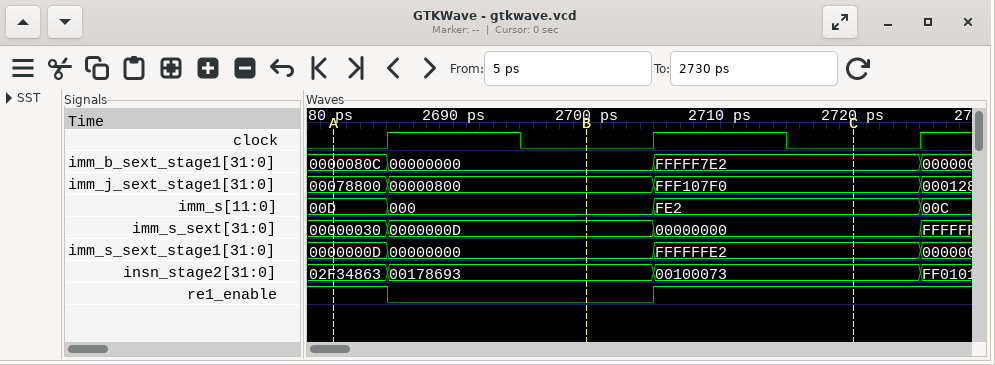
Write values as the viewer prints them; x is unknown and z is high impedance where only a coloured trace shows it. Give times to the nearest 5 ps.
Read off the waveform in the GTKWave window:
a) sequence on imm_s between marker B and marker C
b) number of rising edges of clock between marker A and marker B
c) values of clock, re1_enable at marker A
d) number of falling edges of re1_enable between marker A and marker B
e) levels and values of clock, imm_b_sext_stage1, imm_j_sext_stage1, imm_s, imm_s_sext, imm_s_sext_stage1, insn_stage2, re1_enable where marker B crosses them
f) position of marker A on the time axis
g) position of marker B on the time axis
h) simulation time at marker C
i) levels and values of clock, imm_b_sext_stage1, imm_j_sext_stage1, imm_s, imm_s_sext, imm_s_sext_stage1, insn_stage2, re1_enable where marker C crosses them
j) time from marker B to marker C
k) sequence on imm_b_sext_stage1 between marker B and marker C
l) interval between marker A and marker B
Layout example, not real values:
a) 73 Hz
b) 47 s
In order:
a) 000, FE2
b) 1
c) clock=0, re1_enable=1
d) 1
e) clock=0, imm_b_sext_stage1=00000000, imm_j_sext_stage1=00000800, imm_s=000, imm_s_sext=0000000D, imm_s_sext_stage1=00000000, insn_stage2=00178693, re1_enable=0
f) 2680 ps
g) 2700 ps
h) 2720 ps
i) clock=0, imm_b_sext_stage1=FFFFF7E2, imm_j_sext_stage1=FFF107F0, imm_s=FE2, imm_s_sext=00000000, imm_s_sext_stage1=FFFFFFE2, insn_stage2=00100073, re1_enable=1
j) 20 ps
k) 00000000, FFFFF7E2
l) 20 ps
